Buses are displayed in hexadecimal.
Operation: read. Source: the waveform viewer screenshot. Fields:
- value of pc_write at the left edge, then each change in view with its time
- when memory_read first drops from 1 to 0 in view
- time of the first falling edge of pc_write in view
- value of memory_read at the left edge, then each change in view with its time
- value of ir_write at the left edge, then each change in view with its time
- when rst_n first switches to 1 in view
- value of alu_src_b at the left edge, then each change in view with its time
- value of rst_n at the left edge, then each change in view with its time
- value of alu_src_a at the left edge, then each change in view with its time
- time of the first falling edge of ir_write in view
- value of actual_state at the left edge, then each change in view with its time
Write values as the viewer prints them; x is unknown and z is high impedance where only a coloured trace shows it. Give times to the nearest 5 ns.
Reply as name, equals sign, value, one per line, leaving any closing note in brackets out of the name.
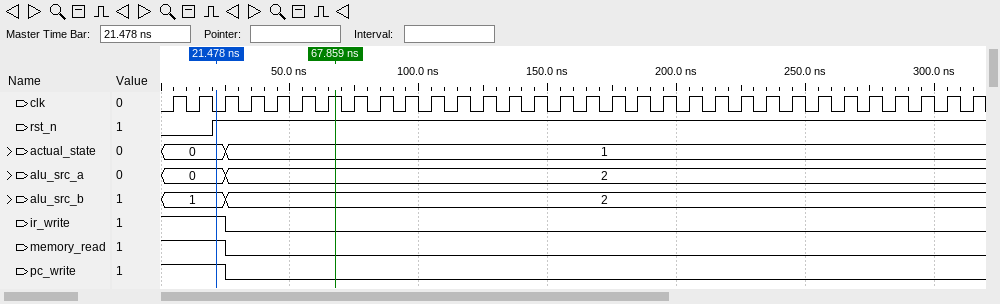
value of pc_write at the left edge, then each change in view with its time = 1, 0 at 25 ns
when memory_read first drops from 1 to 0 in view = 25 ns
time of the first falling edge of pc_write in view = 25 ns
value of memory_read at the left edge, then each change in view with its time = 1, 0 at 25 ns
value of ir_write at the left edge, then each change in view with its time = 1, 0 at 25 ns
when rst_n first switches to 1 in view = 20 ns
value of alu_src_b at the left edge, then each change in view with its time = 1, 2 at 25 ns
value of rst_n at the left edge, then each change in view with its time = 0, 1 at 20 ns
value of alu_src_a at the left edge, then each change in view with its time = 0, 2 at 25 ns
time of the first falling edge of ir_write in view = 25 ns
value of actual_state at the left edge, then each change in view with its time = 0, 1 at 25 ns
